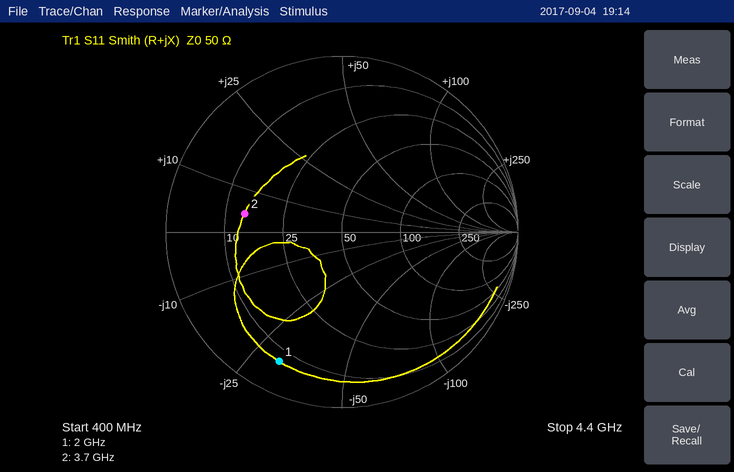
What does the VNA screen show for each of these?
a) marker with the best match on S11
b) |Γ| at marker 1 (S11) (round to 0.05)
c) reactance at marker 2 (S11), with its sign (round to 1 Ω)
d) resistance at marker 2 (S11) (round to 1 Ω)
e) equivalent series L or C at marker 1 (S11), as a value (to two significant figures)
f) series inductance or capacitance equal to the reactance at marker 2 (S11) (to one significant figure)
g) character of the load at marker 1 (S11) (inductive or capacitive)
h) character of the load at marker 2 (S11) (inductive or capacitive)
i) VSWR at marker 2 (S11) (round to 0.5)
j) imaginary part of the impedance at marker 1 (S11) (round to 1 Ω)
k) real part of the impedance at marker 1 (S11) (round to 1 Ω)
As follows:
marker 2
0.80
+4 Ω
14 Ω
2.6 pF
200 pH
capacitive
inductive
3.5
-31 Ω
7 Ω
